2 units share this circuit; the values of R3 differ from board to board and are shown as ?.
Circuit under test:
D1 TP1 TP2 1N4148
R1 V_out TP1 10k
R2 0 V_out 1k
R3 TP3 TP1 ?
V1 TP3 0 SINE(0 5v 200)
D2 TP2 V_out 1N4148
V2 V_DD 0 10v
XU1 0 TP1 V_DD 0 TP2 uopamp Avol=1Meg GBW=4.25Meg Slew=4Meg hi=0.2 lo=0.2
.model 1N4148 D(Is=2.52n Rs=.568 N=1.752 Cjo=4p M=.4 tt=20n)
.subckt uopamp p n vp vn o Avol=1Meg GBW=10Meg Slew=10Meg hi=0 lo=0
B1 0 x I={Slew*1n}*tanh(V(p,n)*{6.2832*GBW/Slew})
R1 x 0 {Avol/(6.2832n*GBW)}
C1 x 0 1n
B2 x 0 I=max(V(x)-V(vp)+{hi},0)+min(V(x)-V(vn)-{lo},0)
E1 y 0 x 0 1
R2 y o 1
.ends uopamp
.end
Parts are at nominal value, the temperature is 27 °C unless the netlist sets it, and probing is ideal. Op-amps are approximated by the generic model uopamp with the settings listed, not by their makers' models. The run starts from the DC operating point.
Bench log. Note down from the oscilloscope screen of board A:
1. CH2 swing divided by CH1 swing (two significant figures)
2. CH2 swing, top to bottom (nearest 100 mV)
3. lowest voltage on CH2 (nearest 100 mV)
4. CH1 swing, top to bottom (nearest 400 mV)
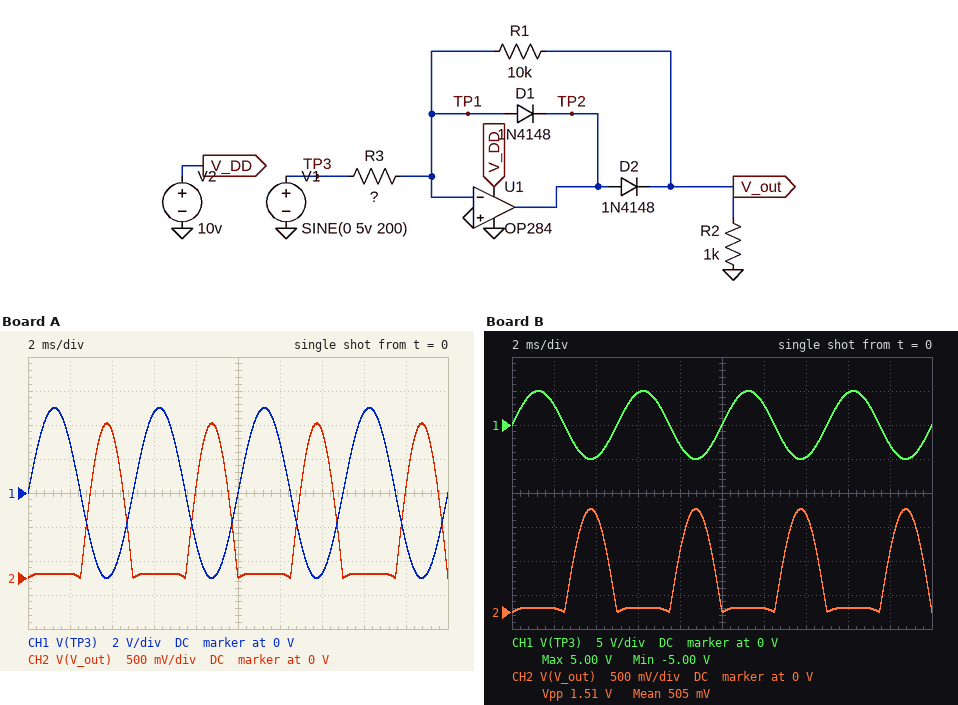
0.23
2.3 V
0 V
10.0 V
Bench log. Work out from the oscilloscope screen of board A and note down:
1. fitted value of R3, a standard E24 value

22 kΩ
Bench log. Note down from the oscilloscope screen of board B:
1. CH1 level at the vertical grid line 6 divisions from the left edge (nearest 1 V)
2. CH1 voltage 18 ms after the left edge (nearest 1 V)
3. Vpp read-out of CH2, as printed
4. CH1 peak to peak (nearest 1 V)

3 V
-3 V
1.51 V
10 V
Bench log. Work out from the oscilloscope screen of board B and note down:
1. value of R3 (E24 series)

33 kΩ
